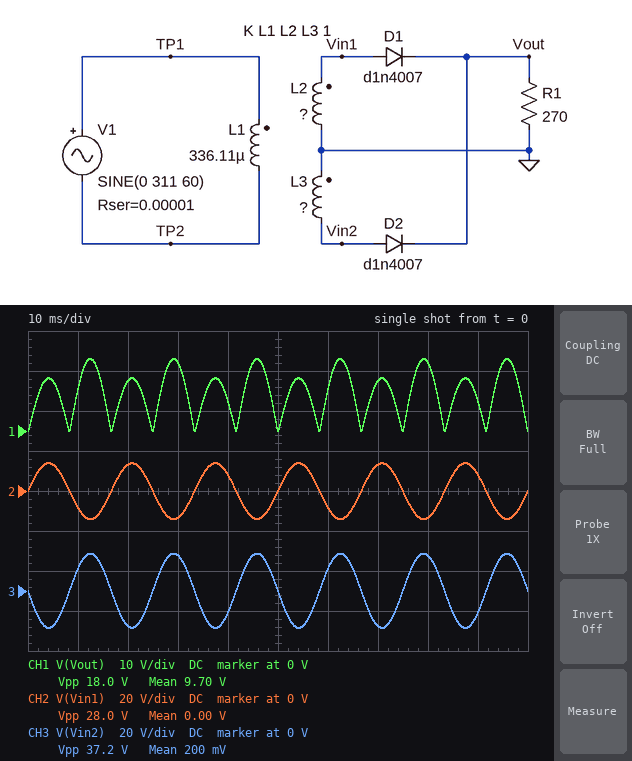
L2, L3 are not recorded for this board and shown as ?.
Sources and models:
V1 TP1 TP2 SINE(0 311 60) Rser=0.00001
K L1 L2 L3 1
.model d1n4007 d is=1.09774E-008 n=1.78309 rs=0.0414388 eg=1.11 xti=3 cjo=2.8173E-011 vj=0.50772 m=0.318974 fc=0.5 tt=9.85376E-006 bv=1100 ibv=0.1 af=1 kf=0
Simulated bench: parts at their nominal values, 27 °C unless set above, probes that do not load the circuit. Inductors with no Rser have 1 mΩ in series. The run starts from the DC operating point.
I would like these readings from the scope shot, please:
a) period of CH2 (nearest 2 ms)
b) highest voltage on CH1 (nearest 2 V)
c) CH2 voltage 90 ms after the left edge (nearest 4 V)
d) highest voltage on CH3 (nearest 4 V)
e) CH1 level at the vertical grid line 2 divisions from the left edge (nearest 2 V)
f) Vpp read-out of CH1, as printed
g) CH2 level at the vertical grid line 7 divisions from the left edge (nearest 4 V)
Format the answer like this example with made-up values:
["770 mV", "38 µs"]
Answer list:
["16 ms", "18 V", "8 V", "20 V", "12 V", "18.0 V", "12 V"]
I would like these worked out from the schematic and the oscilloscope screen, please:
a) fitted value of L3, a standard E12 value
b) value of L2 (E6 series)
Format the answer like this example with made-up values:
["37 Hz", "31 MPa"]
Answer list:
["1.2 µH", "680 nH"]
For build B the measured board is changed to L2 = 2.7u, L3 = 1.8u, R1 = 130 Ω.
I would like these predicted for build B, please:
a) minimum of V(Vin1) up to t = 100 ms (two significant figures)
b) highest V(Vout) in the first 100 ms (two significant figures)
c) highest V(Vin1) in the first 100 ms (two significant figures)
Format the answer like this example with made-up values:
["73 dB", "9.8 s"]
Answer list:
["-28 V", "27 V", "28 V"]
